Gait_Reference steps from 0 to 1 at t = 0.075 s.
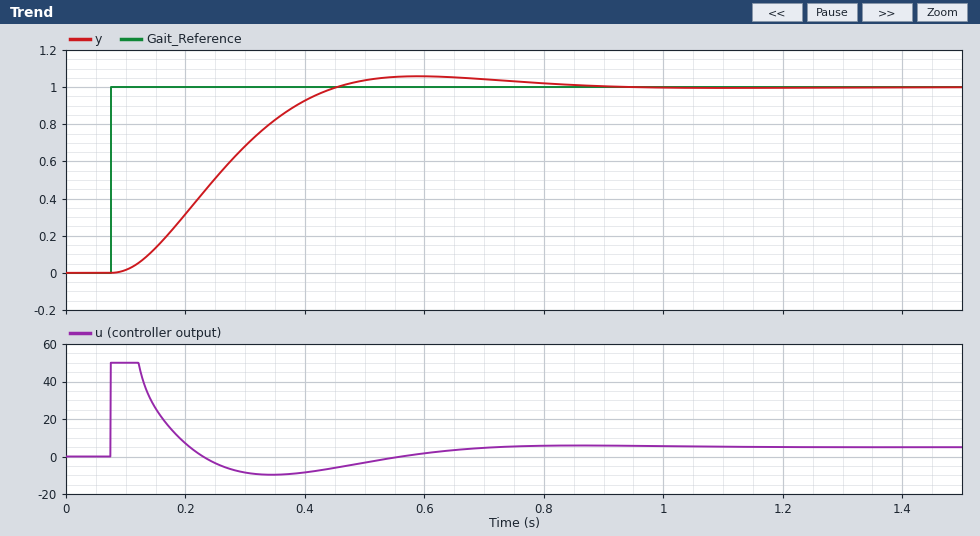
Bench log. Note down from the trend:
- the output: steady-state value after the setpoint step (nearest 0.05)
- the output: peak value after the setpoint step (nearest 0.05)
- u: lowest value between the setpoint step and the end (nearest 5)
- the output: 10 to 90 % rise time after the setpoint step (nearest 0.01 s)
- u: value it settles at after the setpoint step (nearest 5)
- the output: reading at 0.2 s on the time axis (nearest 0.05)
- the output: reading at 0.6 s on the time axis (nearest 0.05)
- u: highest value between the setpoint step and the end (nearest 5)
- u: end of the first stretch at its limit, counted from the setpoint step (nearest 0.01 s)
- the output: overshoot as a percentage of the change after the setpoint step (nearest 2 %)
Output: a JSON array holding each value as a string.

["1.00", "1.05", "-10", "0.25 s", "5", "0.30", "1.05", "50", "0.05 s", "6 %"]
